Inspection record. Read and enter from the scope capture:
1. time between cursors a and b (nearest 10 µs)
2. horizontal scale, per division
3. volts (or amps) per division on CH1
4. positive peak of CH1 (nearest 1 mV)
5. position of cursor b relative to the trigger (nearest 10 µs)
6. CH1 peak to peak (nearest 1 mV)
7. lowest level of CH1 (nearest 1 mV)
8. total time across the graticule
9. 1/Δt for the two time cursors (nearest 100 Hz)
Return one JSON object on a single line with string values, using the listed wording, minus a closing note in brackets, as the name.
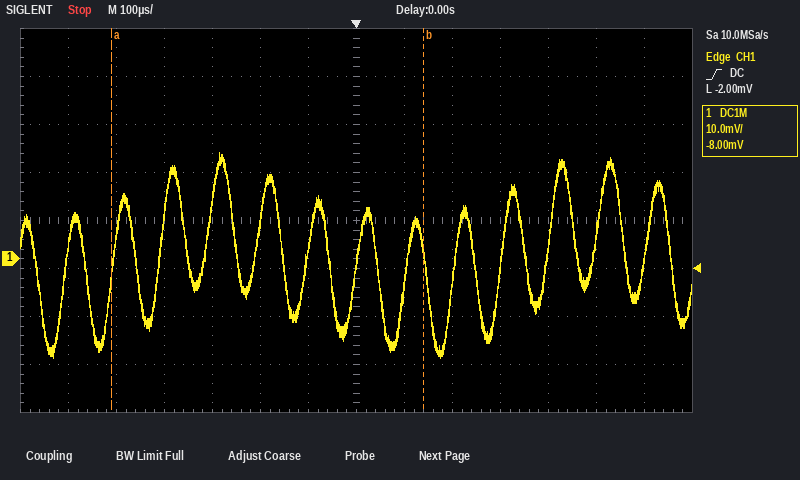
{"time between cursors a and b": "650 µs", "horizontal scale, per division": "100 µs", "volts (or amps) per division on CH1": "10 mV", "positive peak of CH1": "22 mV", "position of cursor b relative to the trigger": "+140 µs", "CH1 peak to peak": "43 mV", "lowest level of CH1": "-21 mV", "total time across the graticule": "1.4 ms", "1/Δt for the two time cursors": "1.5 kHz"}
